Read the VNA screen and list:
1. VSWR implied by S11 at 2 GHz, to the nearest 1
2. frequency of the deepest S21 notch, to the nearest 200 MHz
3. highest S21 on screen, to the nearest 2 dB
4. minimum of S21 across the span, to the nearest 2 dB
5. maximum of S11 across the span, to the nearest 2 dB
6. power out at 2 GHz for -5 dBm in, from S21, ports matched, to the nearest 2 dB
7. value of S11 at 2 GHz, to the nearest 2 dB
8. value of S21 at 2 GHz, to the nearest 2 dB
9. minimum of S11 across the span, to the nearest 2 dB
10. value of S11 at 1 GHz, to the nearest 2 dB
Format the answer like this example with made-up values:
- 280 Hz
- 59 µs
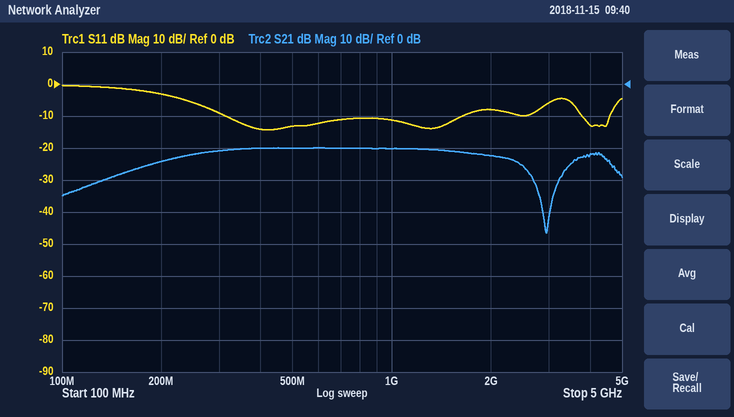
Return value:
- 2
- 3.0 GHz
- -20 dB
- -46 dB
- 0 dB
- -28 dBm
- -8 dB
- -22 dB
- -14 dB
- -12 dB
